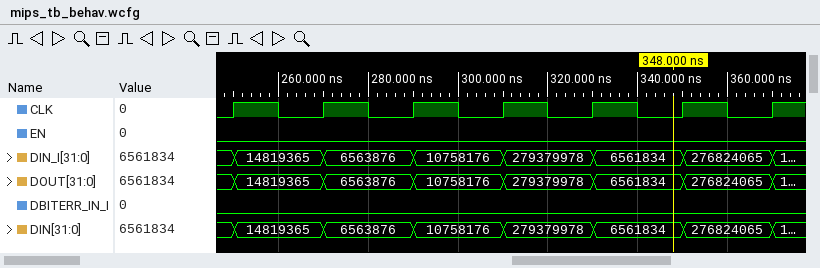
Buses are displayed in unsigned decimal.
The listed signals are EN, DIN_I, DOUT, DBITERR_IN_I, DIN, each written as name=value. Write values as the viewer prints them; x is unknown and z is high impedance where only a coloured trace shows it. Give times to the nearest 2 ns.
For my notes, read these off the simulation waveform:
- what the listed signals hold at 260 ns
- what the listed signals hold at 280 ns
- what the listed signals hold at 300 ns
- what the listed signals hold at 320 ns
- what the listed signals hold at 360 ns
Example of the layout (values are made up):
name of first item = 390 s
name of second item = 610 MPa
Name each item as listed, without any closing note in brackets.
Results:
what the listed signals hold at 260 ns = EN=0, DIN_I=14819365, DOUT=14819365, DBITERR_IN_I=0, DIN=14819365
what the listed signals hold at 280 ns = EN=0, DIN_I=6563876, DOUT=6563876, DBITERR_IN_I=0, DIN=6563876
what the listed signals hold at 300 ns = EN=0, DIN_I=10758176, DOUT=10758176, DBITERR_IN_I=0, DIN=10758176
what the listed signals hold at 320 ns = EN=0, DIN_I=279379978, DOUT=279379978, DBITERR_IN_I=0, DIN=279379978
what the listed signals hold at 360 ns = EN=0, DIN_I=276824065, DOUT=276824065, DBITERR_IN_I=0, DIN=276824065
